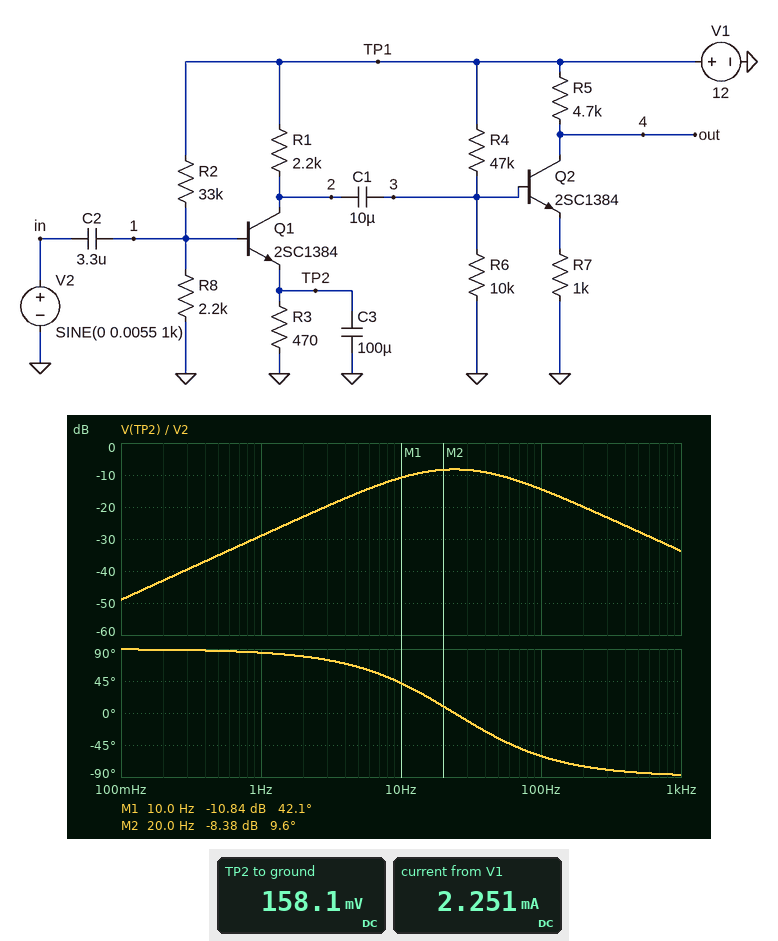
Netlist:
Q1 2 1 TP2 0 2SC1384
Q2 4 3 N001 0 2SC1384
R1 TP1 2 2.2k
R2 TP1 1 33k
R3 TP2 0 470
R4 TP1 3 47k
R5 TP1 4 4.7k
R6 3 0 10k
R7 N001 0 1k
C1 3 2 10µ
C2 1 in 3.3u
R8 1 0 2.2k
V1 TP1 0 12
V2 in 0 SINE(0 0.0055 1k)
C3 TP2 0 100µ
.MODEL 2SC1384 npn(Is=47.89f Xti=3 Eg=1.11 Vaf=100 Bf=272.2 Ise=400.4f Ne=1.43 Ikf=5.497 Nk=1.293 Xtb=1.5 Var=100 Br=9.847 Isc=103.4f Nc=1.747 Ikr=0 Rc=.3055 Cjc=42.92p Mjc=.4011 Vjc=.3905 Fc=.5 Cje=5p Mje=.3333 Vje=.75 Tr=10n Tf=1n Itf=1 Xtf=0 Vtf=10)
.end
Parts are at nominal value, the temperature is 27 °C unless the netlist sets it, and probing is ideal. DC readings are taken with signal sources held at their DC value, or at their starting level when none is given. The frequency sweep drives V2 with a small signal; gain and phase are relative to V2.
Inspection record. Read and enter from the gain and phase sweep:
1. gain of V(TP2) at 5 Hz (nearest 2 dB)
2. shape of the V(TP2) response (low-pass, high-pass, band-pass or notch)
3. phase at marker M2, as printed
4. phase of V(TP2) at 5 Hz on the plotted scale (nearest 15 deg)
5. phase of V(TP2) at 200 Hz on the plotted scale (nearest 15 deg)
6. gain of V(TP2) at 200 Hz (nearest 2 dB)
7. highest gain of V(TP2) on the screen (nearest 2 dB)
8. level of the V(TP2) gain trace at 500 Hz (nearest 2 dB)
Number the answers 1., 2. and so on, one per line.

1. -16 dB
2. band-pass
3. 9.6 deg
4. 60 deg
5. -75 deg
6. -20 dB
7. -8 dB
8. -28 dB
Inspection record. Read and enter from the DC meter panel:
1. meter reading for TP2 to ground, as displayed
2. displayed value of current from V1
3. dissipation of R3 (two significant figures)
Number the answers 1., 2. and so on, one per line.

1. 158.1 mV
2. 2.251 mA
3. 53 µW
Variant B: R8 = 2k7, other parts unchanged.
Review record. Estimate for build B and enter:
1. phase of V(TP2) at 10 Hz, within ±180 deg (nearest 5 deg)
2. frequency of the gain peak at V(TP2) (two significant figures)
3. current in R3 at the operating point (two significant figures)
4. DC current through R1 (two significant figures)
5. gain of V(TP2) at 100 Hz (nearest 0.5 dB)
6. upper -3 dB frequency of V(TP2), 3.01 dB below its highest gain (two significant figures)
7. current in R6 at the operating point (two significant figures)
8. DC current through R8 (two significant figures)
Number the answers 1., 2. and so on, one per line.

1. 45 deg
2. 29 Hz
3. 620 µA
4. 610 µA
5. -9.5 dB
6. 80 Hz
7. 200 µA
8. 330 µA
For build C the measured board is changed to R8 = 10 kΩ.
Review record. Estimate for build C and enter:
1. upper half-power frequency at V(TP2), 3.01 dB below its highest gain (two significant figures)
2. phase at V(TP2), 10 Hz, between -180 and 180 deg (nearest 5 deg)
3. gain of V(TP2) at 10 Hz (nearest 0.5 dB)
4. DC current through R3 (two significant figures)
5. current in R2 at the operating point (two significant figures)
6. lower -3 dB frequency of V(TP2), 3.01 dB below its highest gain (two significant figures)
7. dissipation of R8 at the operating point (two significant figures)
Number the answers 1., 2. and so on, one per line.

1. 300 Hz
2. 30 deg
3. -3.0 dB
4. 4.0 mA
5. 290 µA
6. 5.6 Hz
7. 650 µW
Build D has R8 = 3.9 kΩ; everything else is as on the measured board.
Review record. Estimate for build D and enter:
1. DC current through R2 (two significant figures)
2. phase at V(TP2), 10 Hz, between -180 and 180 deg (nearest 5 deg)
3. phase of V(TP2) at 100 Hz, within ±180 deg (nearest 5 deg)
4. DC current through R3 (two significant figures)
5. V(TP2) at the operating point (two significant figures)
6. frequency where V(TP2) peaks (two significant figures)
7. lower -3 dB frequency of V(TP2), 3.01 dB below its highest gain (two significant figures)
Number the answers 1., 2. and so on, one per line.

1. 330 µA
2. 45 deg
3. -40 deg
4. 1.3 mA
5. 610 mV
6. 34 Hz
7. 9.7 Hz
